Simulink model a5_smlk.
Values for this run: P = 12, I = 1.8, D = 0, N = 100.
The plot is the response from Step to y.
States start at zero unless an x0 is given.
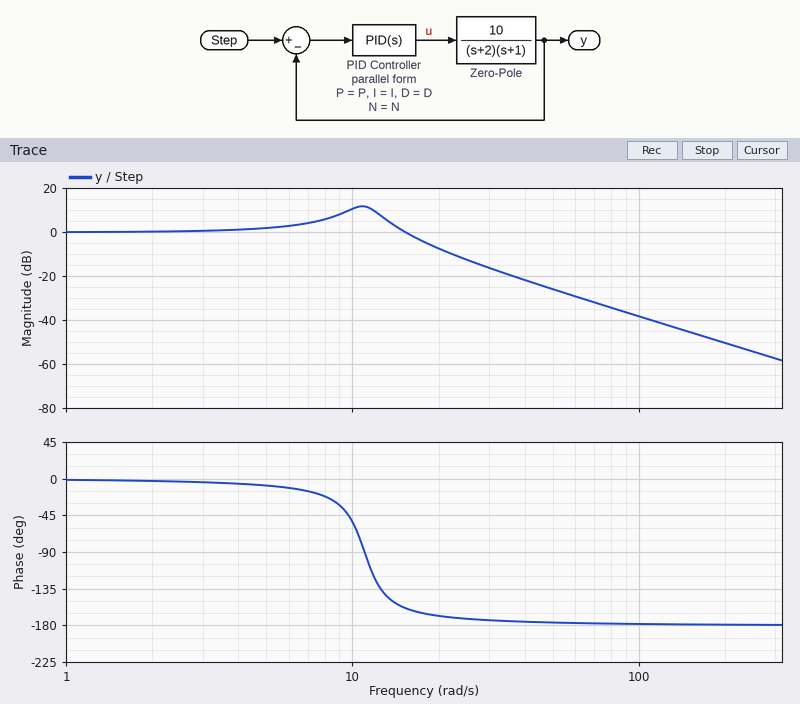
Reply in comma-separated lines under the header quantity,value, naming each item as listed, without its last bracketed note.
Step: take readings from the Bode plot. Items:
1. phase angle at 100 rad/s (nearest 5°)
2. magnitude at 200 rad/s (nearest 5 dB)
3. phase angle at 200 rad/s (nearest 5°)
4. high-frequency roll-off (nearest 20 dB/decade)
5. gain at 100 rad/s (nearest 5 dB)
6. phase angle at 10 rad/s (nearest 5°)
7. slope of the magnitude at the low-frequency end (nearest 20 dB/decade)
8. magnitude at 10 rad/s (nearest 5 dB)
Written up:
quantity,value
phase angle at 100 rad/s,-180°
magnitude at 200 rad/s,-50 dB
phase angle at 200 rad/s,-180°
high-frequency roll-off,-40 dB/decade
gain at 100 rad/s,-40 dB
phase angle at 10 rad/s,-55°
slope of the magnitude at the low-frequency end,0 dB/decade
magnitude at 10 rad/s,10 dB
